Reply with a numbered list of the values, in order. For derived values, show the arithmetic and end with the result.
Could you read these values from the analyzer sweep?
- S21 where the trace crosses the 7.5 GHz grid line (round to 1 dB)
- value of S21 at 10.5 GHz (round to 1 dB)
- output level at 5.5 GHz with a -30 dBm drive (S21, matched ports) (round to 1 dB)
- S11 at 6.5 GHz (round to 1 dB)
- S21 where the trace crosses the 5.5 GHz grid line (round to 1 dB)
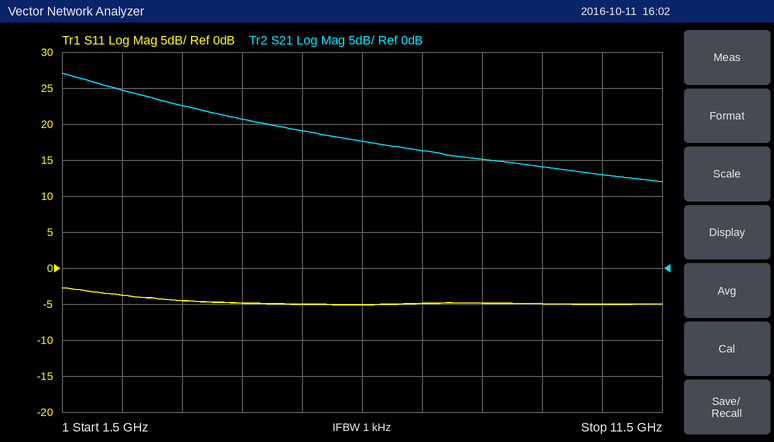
1. 16 dB
2. 13 dB
3. -30 dBm + (19 dB) = -11 dBm
4. -5 dB
5. 19 dB
